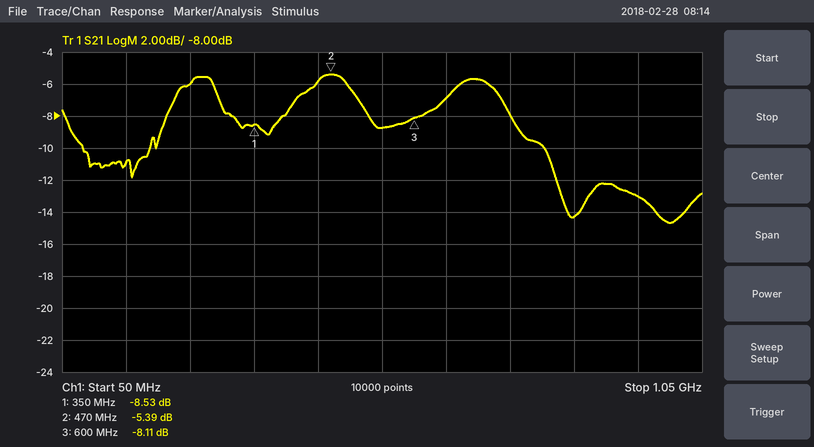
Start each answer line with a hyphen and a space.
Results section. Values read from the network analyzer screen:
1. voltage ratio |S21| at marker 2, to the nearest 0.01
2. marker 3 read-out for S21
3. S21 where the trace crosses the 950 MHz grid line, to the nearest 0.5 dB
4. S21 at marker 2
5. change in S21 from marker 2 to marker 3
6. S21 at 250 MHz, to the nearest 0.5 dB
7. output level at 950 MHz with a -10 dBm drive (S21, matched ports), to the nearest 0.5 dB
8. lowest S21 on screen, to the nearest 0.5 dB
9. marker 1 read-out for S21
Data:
- 0.54
- -8.11 dB
- -13.0 dB
- -5.39 dB
- -2.72 dB
- -6.0 dB
- -23.0 dBm
- -14.5 dB
- -8.53 dB
